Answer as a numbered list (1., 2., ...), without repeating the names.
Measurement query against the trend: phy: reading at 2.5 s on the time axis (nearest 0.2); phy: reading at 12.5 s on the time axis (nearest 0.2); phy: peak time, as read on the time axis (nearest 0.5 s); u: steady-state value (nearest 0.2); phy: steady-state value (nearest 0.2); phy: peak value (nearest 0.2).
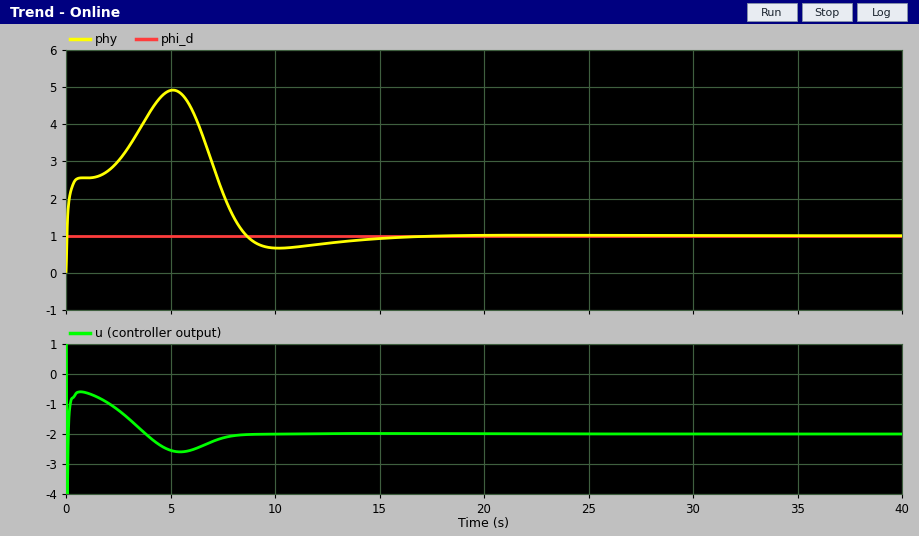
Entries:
1. 3.0
2. 0.8
3. 5.0 s
4. -2.0
5. 1.0
6. 5.0
